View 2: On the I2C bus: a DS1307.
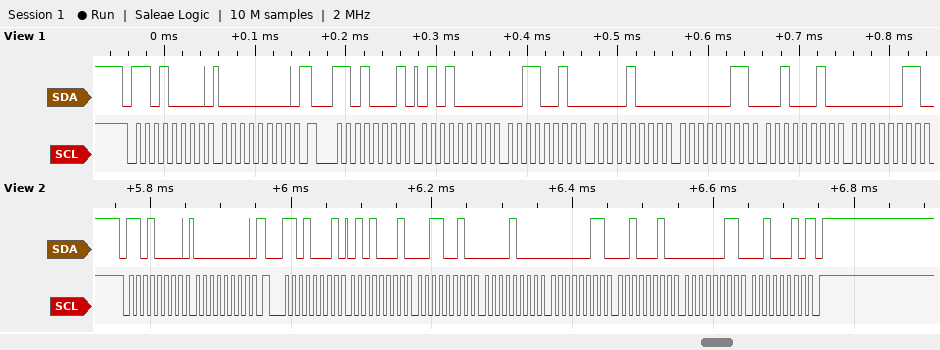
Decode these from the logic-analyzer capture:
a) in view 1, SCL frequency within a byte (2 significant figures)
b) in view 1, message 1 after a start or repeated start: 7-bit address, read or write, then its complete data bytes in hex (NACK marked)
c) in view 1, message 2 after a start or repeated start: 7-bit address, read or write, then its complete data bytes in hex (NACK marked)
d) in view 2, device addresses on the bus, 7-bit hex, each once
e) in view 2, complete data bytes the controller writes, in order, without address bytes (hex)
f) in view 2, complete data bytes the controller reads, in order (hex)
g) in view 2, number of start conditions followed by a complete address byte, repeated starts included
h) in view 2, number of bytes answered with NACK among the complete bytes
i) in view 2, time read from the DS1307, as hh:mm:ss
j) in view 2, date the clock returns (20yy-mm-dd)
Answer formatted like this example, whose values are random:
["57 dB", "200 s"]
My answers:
["100 kHz", "0x68 write: 00", "0x68 read: 50 32 08 03 22 03", "0x68", "00", "51 32 08 03 22 03 22", "2", "1", "08:32:51", "2022-03-22"]
